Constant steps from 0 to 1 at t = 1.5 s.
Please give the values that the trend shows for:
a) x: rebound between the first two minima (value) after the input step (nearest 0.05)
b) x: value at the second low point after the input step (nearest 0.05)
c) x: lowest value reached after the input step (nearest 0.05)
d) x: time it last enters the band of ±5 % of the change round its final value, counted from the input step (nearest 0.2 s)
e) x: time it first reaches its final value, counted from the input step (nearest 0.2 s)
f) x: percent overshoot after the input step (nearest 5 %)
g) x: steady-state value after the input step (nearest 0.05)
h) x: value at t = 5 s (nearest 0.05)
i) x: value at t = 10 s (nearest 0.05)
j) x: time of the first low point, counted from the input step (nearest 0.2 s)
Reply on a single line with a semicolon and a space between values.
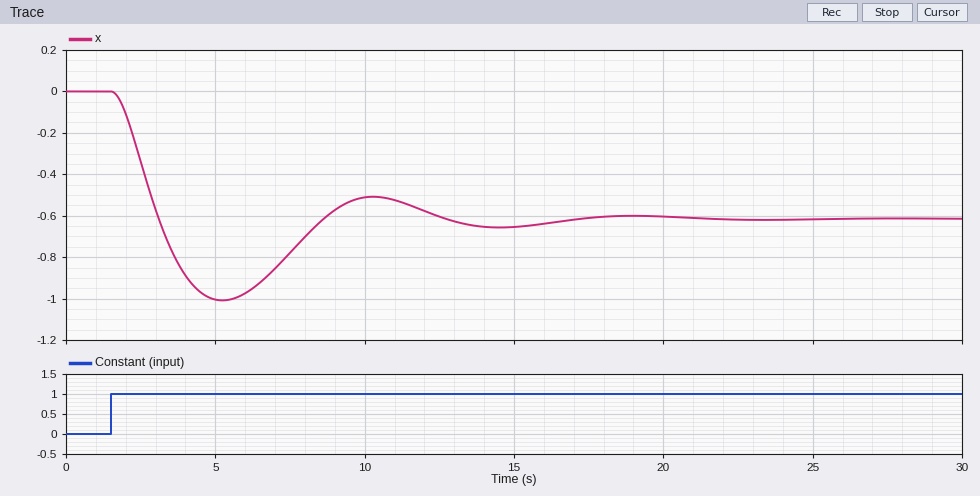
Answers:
-0.50; -0.65; -1.00; 14.2 s; 1.6 s; 65 %; -0.60; -1.00; -0.50; 3.8 s
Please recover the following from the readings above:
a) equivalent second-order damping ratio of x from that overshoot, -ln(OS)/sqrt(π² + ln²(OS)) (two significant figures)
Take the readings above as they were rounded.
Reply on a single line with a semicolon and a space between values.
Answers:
0.14
